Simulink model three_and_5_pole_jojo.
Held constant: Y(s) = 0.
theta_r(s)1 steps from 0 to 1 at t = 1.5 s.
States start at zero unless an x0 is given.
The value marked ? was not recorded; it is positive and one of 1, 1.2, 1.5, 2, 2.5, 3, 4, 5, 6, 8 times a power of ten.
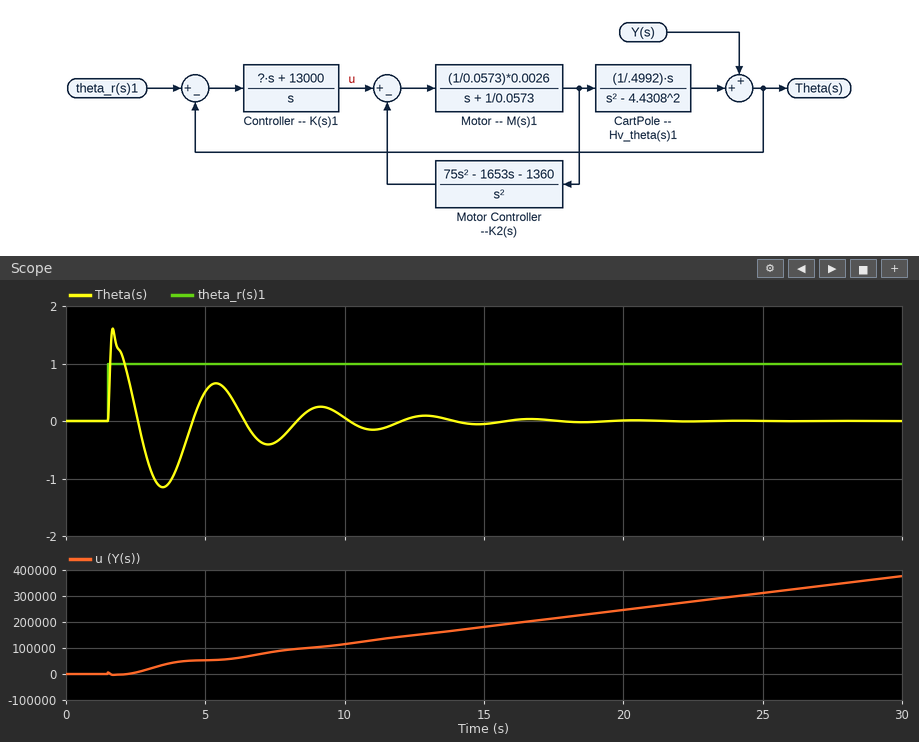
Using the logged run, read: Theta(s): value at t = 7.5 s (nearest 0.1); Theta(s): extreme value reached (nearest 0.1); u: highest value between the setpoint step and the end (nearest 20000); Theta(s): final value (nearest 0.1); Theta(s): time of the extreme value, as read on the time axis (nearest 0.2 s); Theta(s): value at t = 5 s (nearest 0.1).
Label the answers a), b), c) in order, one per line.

a) -0.4
b) 1.6
c) 380000
d) 0.0
e) 1.6 s
f) 0.5
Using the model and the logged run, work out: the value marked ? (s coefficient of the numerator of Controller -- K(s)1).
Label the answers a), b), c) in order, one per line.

a) 6000
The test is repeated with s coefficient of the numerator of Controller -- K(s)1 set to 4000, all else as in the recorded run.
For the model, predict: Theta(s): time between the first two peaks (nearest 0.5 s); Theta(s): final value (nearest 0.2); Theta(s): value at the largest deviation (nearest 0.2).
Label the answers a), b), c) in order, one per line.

a) 3.0 s
b) 0.0
c) 1.8
